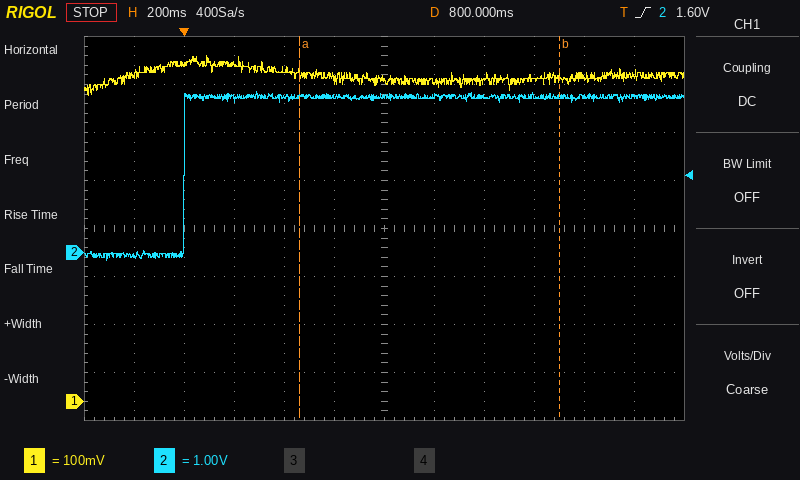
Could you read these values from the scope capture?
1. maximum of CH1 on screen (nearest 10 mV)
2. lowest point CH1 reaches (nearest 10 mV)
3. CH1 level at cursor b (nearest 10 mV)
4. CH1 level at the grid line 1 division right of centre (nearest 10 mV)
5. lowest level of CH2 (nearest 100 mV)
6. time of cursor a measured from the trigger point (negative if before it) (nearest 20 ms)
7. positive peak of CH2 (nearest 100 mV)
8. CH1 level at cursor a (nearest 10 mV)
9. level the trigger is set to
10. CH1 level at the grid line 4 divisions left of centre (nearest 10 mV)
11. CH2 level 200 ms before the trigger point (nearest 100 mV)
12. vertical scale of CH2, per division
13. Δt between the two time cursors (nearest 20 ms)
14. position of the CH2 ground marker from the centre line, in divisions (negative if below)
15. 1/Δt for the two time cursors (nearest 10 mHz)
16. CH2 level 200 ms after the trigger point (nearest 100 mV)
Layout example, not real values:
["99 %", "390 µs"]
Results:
["720 mV", "640 mV", "670 mV", "670 mV", "-200 mV", "+460 ms", "3.4 V", "680 mV", "1.60 V", "700 mV", "-100 mV", "1 V", "1.04 s", "-0.5 div", "960 mHz", "3.2 V"]
